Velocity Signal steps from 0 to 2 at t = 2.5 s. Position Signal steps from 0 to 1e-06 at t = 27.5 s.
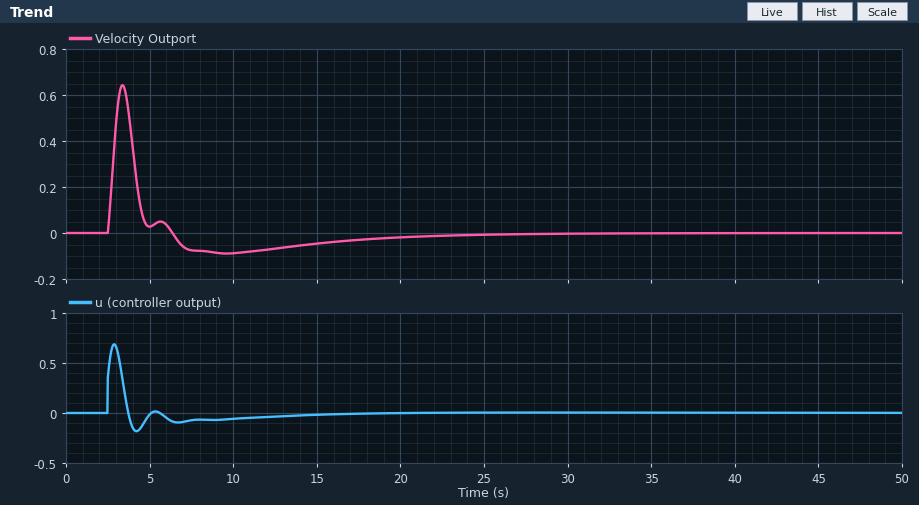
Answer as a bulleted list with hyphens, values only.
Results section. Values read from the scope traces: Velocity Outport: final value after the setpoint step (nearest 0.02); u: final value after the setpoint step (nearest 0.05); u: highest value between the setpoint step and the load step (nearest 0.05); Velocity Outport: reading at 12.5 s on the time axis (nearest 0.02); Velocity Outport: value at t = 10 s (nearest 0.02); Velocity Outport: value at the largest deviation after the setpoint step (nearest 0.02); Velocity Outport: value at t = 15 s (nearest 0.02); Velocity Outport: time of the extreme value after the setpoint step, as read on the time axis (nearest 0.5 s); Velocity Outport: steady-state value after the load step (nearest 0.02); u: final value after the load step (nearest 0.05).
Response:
- 0.00
- 0.00
- 0.70
- -0.06
- -0.08
- 0.64
- -0.04
- 3.5 s
- 0.00
- 0.00
